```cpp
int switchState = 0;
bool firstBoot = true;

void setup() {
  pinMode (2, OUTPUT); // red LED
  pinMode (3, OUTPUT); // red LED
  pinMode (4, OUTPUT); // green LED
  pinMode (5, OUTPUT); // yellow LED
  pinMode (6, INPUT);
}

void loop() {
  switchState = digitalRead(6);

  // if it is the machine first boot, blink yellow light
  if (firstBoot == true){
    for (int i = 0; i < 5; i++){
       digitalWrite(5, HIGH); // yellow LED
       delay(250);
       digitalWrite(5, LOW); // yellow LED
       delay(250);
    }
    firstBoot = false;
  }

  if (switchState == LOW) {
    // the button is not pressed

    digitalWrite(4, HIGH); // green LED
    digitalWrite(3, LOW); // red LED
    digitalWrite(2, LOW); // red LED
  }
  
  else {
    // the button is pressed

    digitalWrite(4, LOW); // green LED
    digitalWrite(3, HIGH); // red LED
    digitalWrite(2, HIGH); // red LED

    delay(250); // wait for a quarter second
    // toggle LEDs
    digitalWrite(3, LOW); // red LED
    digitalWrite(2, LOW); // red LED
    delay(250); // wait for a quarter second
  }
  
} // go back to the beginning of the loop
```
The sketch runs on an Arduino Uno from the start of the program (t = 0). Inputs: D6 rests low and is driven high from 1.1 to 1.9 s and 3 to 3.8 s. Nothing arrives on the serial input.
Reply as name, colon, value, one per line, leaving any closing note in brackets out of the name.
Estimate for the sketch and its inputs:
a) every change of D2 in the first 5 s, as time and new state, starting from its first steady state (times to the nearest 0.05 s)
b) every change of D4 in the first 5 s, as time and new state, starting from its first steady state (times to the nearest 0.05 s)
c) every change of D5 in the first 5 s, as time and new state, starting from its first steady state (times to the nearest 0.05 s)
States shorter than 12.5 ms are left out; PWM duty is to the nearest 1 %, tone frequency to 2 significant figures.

every change of D2 in the first 5 s, as time and new state, starting from its first steady state: 0 s low; 3 s high; 3.25 s low; 3.5 s high; 3.75 s low
every change of D4 in the first 5 s, as time and new state, starting from its first steady state: 0 s low; 2.5 s high; 3 s low; 4 s high
every change of D5 in the first 5 s, as time and new state, starting from its first steady state: 0 s high; 0.25 s low; 0.5 s high; 0.75 s low; 1 s high; 1.25 s low; 1.5 s high; 1.75 s low; 2 s high; 2.25 s low
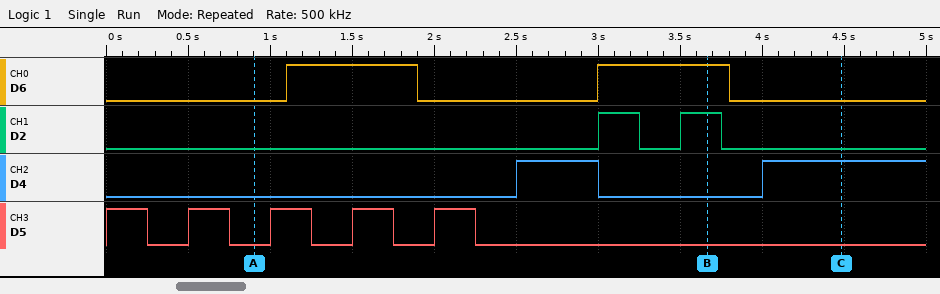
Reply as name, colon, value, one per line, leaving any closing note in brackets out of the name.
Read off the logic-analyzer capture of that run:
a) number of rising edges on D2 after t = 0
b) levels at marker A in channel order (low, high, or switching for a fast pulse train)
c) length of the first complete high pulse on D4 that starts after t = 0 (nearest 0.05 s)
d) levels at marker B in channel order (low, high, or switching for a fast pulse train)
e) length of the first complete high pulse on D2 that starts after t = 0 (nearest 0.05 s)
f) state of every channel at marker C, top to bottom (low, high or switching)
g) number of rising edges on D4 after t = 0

number of rising edges on D2 after t = 0: 2
levels at marker A in channel order: D6 low, D2 low, D4 low, D5 low
length of the first complete high pulse on D4 that starts after t = 0: 0.50 s
levels at marker B in channel order: D6 high, D2 high, D4 low, D5 low
length of the first complete high pulse on D2 that starts after t = 0: 0.25 s
state of every channel at marker C, top to bottom: D6 low, D2 low, D4 high, D5 low
number of rising edges on D4 after t = 0: 2
